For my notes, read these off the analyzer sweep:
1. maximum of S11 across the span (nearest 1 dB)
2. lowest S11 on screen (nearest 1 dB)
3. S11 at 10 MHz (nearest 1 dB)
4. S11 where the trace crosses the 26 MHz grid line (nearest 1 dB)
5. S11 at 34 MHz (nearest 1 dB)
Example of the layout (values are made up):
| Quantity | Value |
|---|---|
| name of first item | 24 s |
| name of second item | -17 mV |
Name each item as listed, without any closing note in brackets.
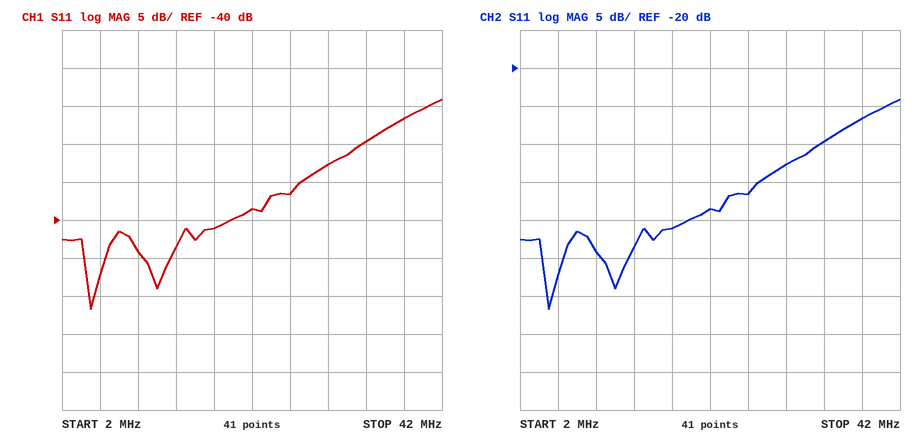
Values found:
| Quantity | Value |
|---|---|
| maximum of S11 across the span | -24 dB |
| lowest S11 on screen | -52 dB |
| S11 at 10 MHz | -44 dB |
| S11 where the trace crosses the 26 MHz grid line | -37 dB |
| S11 at 34 MHz | -30 dB |
